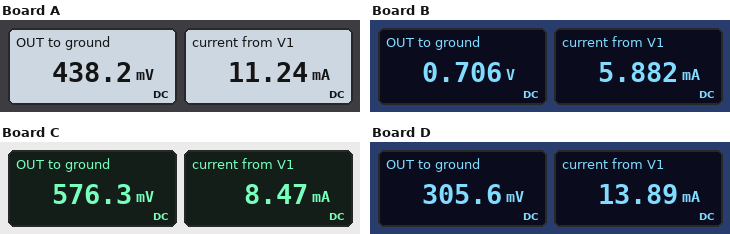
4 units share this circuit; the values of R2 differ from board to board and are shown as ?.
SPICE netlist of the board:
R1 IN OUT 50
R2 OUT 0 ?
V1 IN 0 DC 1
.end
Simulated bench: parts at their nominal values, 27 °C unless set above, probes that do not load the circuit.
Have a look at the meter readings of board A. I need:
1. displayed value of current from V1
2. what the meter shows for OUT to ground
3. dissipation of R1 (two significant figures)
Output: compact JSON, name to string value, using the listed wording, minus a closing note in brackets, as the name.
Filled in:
{"displayed value of current from V1": "11.24 mA", "what the meter shows for OUT to ground": "438.2 mV", "dissipation of R1": "6.3 mW"}
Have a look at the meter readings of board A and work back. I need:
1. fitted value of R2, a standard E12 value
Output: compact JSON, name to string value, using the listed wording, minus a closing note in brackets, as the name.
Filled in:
{"fitted value of R2, a standard E12 value": "39 Ω"}
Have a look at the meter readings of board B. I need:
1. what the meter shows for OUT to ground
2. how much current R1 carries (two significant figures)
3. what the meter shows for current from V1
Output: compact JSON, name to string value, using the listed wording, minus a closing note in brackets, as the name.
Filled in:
{"what the meter shows for OUT to ground": "0.706 V", "how much current R1 carries": "5.9 mA", "what the meter shows for current from V1": "5.882 mA"}
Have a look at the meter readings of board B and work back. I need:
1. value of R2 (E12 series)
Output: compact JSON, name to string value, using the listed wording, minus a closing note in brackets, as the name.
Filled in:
{"value of R2": "120 Ω"}
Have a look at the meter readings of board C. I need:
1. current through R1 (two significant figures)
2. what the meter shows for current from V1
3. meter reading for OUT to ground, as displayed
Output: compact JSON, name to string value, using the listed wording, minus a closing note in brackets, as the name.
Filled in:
{"current through R1": "8.5 mA", "what the meter shows for current from V1": "8.47 mA", "meter reading for OUT to ground, as displayed": "576.3 mV"}
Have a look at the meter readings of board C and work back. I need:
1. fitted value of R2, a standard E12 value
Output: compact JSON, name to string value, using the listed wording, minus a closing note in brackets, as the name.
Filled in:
{"fitted value of R2, a standard E12 value": "68 Ω"}
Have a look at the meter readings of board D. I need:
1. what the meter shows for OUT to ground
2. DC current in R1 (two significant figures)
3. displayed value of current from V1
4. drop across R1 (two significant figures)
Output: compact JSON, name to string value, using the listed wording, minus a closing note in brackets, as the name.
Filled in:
{"what the meter shows for OUT to ground": "305.6 mV", "DC current in R1": "14 mA", "displayed value of current from V1": "13.89 mA", "drop across R1": "690 mV"}
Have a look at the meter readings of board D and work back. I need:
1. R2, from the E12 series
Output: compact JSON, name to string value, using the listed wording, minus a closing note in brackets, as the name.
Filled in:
{"R2, from the E12 series": "22 Ω"}
